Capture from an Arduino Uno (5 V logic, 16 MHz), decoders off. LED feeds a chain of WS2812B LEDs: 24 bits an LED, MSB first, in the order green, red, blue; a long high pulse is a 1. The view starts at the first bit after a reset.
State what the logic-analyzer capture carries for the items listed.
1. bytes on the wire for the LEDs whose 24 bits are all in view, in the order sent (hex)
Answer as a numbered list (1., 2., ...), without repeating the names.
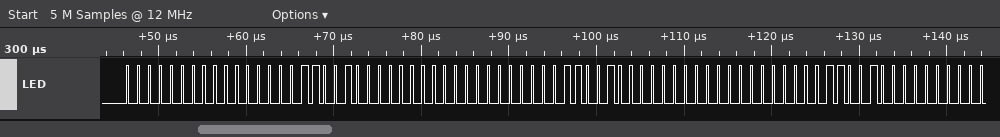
1. 00 00 C8 00 00 C8 00 00 C8
